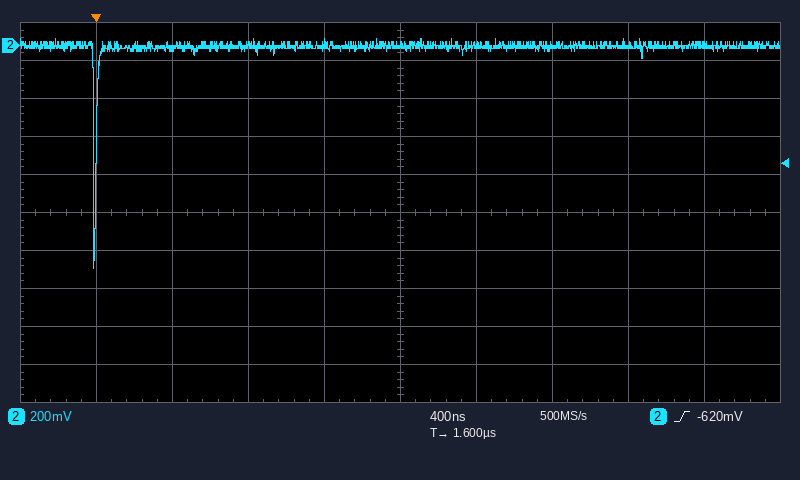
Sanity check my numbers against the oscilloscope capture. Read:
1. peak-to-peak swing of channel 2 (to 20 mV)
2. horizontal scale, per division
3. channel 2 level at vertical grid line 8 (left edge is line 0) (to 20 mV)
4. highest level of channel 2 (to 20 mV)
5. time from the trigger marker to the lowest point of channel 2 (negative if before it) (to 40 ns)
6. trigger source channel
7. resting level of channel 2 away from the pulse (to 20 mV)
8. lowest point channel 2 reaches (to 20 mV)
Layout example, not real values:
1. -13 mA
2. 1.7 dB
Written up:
1. 1.22 V
2. 400 ns
3. 0 mV
4. 40 mV
5. 0 ns
6. channel 2
7. 0 mV
8. -1.18 V
